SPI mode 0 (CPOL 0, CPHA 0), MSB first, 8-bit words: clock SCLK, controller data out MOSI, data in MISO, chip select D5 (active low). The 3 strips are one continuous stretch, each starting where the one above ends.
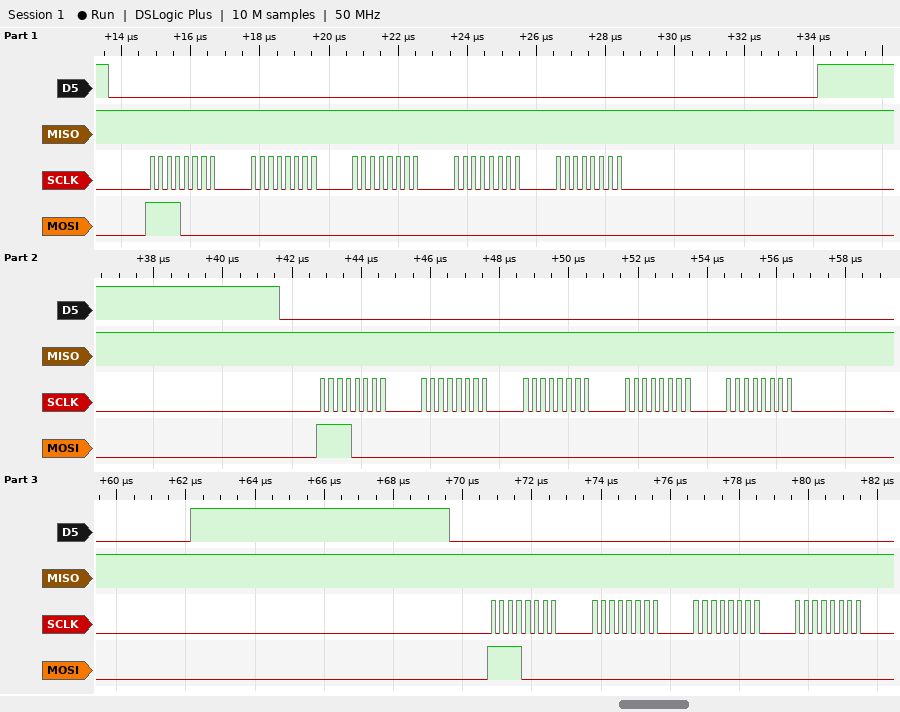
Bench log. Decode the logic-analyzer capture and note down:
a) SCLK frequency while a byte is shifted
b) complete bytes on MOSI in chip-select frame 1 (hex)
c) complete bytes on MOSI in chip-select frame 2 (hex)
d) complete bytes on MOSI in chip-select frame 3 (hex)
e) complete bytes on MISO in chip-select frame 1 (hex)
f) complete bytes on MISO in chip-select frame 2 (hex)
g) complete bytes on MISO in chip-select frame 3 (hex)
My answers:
4 MHz
F0 00 00 00 00
F0 00 00 00 00
F0 00 00 00
FF FF FF FF FF
FF FF FF FF FF
FF FF FF FF
